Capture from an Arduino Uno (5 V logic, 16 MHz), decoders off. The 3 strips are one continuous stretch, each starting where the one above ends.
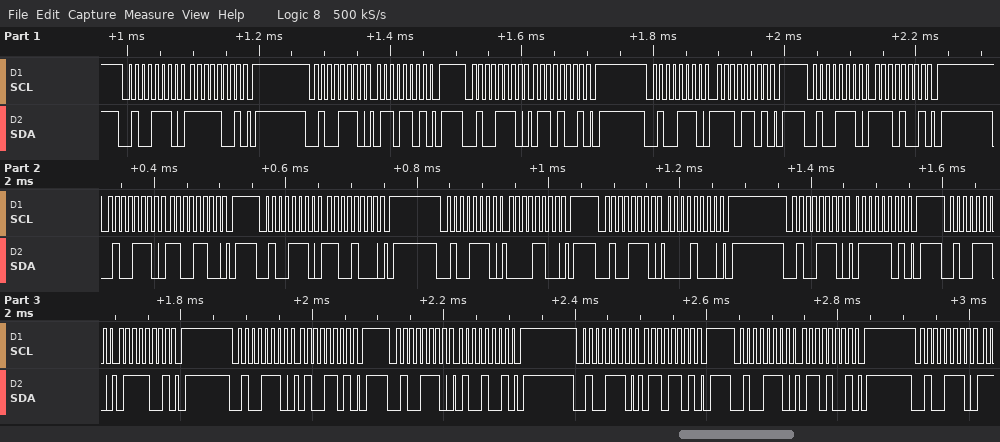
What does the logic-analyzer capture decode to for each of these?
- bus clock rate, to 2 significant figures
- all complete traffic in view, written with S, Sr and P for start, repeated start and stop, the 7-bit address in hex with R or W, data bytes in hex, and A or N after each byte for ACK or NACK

100 kHz
S 27W A F9 A P S 27W A 6D A P S 27W A 69 A P S 27W A ED A P S 27W A E9 A P S 27W A CC A P S 27W A C8 A P S 27W A 0C A P S 27W A 08 A P S 27W A 7D A P S 27W A 79 A P S 27W A 4D A P S 27W A 49 A P S 27W A 6D A P S 27W A 69 A P S 27W A
